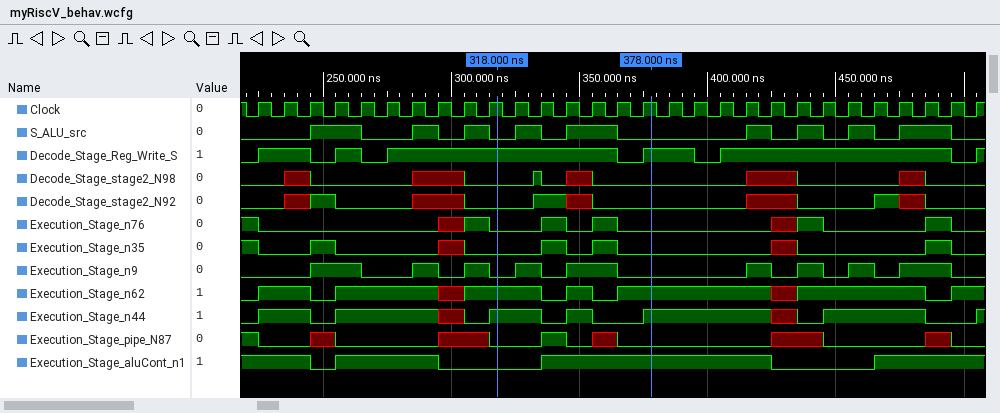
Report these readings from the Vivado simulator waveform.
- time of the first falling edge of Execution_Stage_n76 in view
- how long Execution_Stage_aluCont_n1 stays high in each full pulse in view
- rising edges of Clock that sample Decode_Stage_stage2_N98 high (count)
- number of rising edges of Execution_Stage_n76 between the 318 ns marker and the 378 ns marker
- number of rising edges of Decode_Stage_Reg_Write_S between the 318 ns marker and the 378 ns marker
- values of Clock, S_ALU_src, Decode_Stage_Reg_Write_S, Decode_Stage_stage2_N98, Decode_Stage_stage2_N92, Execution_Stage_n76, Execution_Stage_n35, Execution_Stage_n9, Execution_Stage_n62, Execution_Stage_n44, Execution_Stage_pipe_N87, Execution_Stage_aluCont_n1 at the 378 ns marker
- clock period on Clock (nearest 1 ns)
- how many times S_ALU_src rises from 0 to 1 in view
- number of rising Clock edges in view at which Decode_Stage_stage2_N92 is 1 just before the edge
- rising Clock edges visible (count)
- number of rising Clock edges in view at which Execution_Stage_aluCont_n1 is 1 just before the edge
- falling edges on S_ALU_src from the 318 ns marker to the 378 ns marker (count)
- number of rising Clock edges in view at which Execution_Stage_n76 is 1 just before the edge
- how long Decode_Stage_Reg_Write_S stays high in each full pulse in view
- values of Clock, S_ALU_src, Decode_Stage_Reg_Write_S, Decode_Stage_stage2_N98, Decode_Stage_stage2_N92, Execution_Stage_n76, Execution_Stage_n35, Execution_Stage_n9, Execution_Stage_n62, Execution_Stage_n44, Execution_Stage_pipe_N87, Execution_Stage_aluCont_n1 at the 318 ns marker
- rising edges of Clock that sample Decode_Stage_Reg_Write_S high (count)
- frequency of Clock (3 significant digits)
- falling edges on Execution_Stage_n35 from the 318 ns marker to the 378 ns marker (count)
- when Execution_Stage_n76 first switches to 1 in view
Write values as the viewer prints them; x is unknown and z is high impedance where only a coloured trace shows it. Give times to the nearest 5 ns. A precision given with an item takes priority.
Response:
225 ns
40 ns, 90 ns
1
2
1
Clock=1, S_ALU_src=0, Decode_Stage_Reg_Write_S=1, Decode_Stage_stage2_N98=0, Decode_Stage_stage2_N92=0, Execution_Stage_n76=0, Execution_Stage_n35=0, Execution_Stage_n9=0, Execution_Stage_n62=1, Execution_Stage_n44=1, Execution_Stage_pipe_N87=0, Execution_Stage_aluCont_n1=1
10 ns
9
4
29
20
2
6
20 ns, 10 ns, 90 ns, 20 ns, 90 ns
Clock=1, S_ALU_src=0, Decode_Stage_Reg_Write_S=1, Decode_Stage_stage2_N98=0, Decode_Stage_stage2_N92=0, Execution_Stage_n76=0, Execution_Stage_n35=0, Execution_Stage_n9=0, Execution_Stage_n62=1, Execution_Stage_n44=1, Execution_Stage_pipe_N87=0, Execution_Stage_aluCont_n1=0
23
100 MHz
2
305 ns
